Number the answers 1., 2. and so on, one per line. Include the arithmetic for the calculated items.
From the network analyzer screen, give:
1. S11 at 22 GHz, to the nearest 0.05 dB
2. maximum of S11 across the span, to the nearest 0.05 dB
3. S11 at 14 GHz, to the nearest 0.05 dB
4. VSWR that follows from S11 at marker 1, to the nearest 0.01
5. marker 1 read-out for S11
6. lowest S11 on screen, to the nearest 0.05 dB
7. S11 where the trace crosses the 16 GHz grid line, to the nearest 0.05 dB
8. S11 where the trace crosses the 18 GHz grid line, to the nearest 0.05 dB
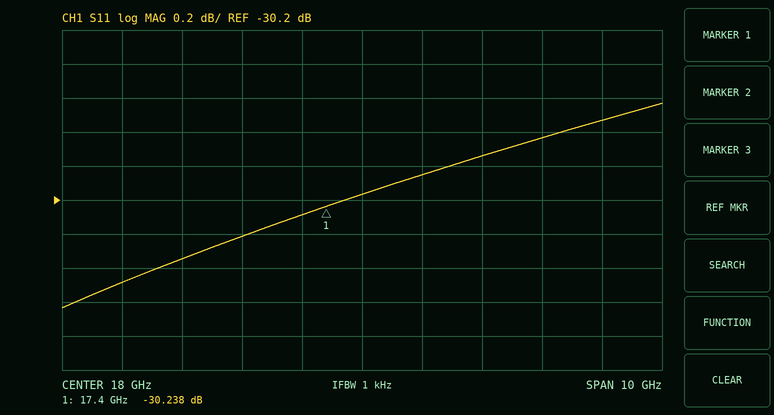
1. -29.75 dB
2. -29.65 dB
3. -30.70 dB
4. (1 + 0.0308)/(1 − 0.0308) ≈ 1.06
5. -30.238 dB
6. -30.85 dB
7. -30.40 dB
8. -30.15 dB
